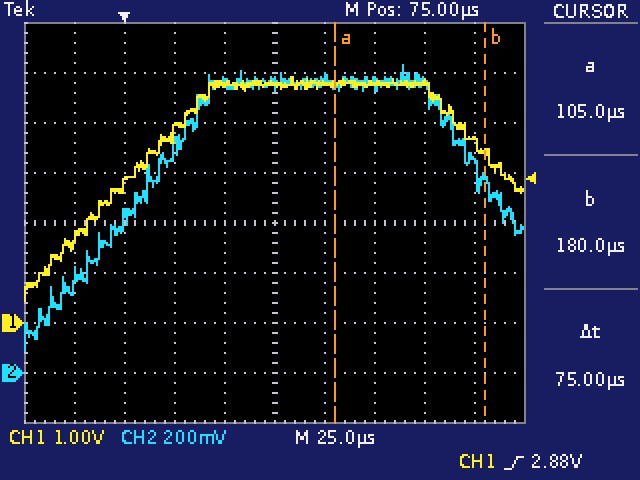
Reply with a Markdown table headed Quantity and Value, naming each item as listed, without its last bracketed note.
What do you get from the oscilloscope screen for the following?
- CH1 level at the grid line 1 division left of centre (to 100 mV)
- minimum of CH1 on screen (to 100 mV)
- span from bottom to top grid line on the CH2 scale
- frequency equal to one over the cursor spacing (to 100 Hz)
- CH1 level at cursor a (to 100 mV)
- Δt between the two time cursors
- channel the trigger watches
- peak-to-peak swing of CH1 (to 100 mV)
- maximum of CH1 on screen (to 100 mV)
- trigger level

| Quantity | Value |
|---|---|
| CH1 level at the grid line 1 division left of centre | 4.8 V |
| minimum of CH1 on screen | 400 mV |
| span from bottom to top grid line on the CH2 scale | 1.6 V |
| frequency equal to one over the cursor spacing | 13.3 kHz |
| CH1 level at cursor a | 4.8 V |
| Δt between the two time cursors | 75 µs |
| channel the trigger watches | CH1 |
| peak-to-peak swing of CH1 | 4.5 V |
| maximum of CH1 on screen | 4.9 V |
| trigger level | 2.88 V |
